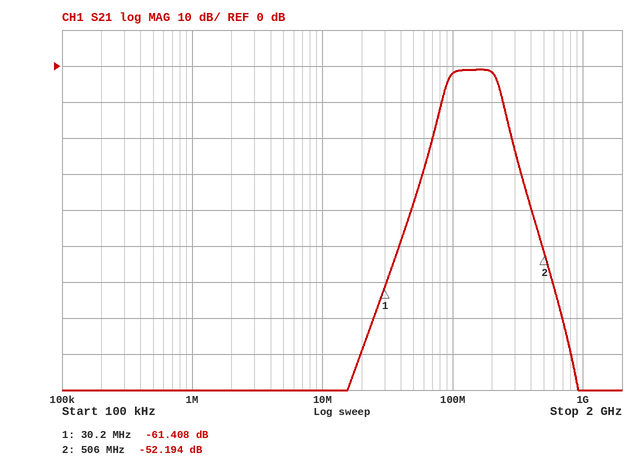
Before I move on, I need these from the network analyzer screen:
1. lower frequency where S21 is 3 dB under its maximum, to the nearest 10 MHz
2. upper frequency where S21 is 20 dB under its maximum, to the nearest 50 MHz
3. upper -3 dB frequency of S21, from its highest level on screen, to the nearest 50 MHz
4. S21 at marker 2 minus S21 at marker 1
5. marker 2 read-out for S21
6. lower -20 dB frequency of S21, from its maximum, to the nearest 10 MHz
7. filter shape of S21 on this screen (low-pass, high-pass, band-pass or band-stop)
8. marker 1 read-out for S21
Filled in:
90 MHz
300 MHz
200 MHz
9.214 dB
-52.194 dB
70 MHz
band-pass
-61.408 dB
